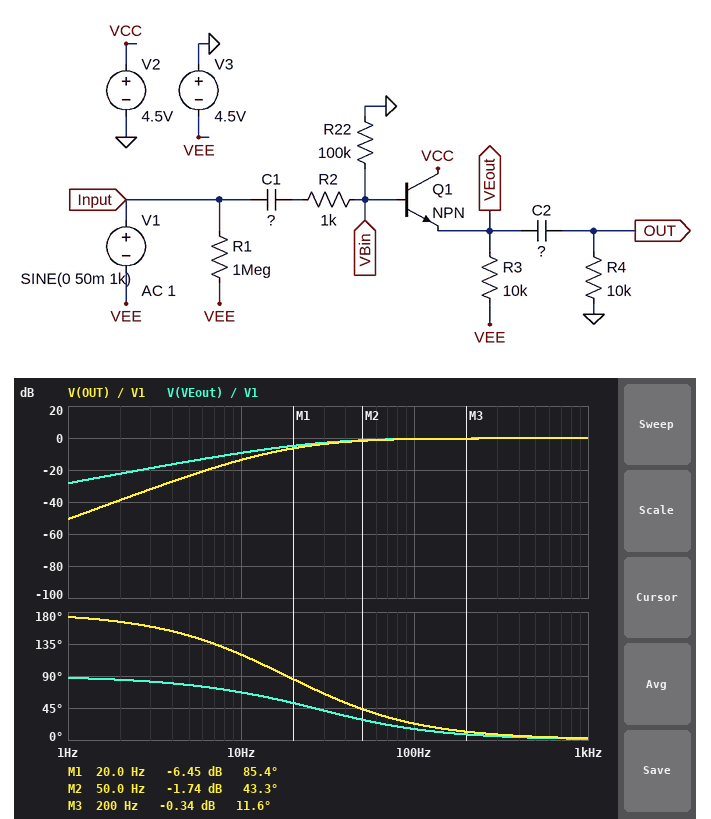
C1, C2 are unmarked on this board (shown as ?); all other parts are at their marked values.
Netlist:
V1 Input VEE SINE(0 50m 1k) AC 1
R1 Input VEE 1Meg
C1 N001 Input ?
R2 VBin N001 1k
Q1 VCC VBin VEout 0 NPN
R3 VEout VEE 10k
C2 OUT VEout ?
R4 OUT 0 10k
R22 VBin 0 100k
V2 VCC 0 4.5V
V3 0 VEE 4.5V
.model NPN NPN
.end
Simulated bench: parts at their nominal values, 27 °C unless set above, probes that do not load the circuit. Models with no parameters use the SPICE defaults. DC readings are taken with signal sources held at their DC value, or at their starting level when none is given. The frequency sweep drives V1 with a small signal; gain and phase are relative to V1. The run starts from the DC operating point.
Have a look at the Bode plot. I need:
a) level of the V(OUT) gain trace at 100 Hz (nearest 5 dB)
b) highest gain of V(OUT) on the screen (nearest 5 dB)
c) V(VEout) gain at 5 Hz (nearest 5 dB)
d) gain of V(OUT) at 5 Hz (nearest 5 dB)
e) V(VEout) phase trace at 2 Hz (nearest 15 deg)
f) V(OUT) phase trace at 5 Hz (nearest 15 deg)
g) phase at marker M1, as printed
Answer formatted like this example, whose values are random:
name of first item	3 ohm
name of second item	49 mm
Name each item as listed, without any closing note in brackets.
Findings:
level of the V(OUT) gain trace at 100 Hz	0 dB
highest gain of V(OUT) on the screen	0 dB
V(VEout) gain at 5 Hz	-15 dB
gain of V(OUT) at 5 Hz	-25 dB
V(VEout) phase trace at 2 Hz	90 deg
V(OUT) phase trace at 5 Hz	150 deg
phase at marker M1, as printed	85.4 deg
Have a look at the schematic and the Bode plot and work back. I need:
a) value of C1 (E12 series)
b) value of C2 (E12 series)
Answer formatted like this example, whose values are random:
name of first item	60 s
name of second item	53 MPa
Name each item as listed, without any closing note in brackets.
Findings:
value of C1	68 nF
value of C2	1.2 µF
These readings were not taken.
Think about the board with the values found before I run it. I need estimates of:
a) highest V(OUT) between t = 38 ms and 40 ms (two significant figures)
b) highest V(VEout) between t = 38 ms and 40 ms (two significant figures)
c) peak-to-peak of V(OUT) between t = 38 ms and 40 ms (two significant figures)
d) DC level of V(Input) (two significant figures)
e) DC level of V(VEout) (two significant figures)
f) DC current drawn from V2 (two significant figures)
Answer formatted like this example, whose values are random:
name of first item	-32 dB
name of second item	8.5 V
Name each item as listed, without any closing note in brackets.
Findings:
highest V(OUT) between t = 38 ms and 40 ms	49 mV
highest V(VEout) between t = 38 ms and 40 ms	-1.0 V
peak-to-peak of V(OUT) between t = 38 ms and 40 ms	97 mV
DC level of V(Input)	-4.5 V
DC level of V(VEout)	-1.1 V
DC current drawn from V2	340 µA
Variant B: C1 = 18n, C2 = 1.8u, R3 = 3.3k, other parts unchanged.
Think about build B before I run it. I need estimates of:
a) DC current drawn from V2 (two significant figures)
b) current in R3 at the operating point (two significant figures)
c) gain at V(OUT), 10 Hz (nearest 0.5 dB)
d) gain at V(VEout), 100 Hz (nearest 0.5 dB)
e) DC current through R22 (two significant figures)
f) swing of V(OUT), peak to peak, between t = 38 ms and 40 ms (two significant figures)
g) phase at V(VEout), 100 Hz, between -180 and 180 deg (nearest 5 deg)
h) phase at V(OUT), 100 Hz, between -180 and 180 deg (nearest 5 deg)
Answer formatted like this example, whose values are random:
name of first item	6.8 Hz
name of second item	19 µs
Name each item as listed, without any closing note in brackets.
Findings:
DC current drawn from V2	860 µA
current in R3 at the operating point	870 µA
gain at V(OUT), 10 Hz	-24.0 dB
gain at V(VEout), 100 Hz	-4.0 dB
DC current through R22	8.6 µA
swing of V(OUT), peak to peak, between t = 38 ms and 40 ms	97 mV
phase at V(VEout), 100 Hz, between -180 and 180 deg	50 deg
phase at V(OUT), 100 Hz, between -180 and 180 deg	55 deg
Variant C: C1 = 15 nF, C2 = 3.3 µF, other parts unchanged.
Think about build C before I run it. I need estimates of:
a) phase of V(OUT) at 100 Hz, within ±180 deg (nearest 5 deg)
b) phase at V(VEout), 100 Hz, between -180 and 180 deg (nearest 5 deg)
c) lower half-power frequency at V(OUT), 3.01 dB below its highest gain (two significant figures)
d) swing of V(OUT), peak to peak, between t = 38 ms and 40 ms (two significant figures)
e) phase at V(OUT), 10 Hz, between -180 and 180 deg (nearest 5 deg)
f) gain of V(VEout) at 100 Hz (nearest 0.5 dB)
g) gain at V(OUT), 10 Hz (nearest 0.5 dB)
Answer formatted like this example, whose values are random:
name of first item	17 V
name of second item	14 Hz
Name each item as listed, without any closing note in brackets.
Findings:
phase of V(OUT) at 100 Hz, within ±180 deg	55 deg
phase at V(VEout), 100 Hz, between -180 and 180 deg	50 deg
lower half-power frequency at V(OUT), 3.01 dB below its highest gain	130 Hz
swing of V(OUT), peak to peak, between t = 38 ms and 40 ms	97 mV
phase at V(OUT), 10 Hz, between -180 and 180 deg	110 deg
gain of V(VEout) at 100 Hz	-4.5 dB
gain at V(OUT), 10 Hz	-23.0 dB
